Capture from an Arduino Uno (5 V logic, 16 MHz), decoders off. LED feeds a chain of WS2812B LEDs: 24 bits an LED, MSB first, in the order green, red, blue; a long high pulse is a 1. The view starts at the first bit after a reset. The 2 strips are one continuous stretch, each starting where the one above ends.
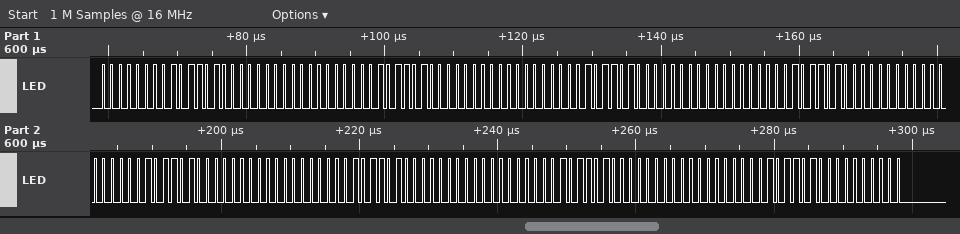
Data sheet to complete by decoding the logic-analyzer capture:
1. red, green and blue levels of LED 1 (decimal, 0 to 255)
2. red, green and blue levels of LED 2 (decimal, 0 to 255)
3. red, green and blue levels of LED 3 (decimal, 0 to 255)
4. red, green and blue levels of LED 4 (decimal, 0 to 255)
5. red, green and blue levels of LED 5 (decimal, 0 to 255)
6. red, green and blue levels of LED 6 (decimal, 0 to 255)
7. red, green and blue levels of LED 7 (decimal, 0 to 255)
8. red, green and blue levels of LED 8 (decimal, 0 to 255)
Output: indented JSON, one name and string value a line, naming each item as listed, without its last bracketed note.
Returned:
{
  "red, green and blue levels of LED 1": "180, 0, 0",
  "red, green and blue levels of LED 2": "180, 0, 0",
  "red, green and blue levels of LED 3": "180, 0, 0",
  "red, green and blue levels of LED 4": "180, 0, 0",
  "red, green and blue levels of LED 5": "180, 0, 0",
  "red, green and blue levels of LED 6": "180, 0, 0",
  "red, green and blue levels of LED 7": "180, 0, 0",
  "red, green and blue levels of LED 8": "180, 0, 0"
}
